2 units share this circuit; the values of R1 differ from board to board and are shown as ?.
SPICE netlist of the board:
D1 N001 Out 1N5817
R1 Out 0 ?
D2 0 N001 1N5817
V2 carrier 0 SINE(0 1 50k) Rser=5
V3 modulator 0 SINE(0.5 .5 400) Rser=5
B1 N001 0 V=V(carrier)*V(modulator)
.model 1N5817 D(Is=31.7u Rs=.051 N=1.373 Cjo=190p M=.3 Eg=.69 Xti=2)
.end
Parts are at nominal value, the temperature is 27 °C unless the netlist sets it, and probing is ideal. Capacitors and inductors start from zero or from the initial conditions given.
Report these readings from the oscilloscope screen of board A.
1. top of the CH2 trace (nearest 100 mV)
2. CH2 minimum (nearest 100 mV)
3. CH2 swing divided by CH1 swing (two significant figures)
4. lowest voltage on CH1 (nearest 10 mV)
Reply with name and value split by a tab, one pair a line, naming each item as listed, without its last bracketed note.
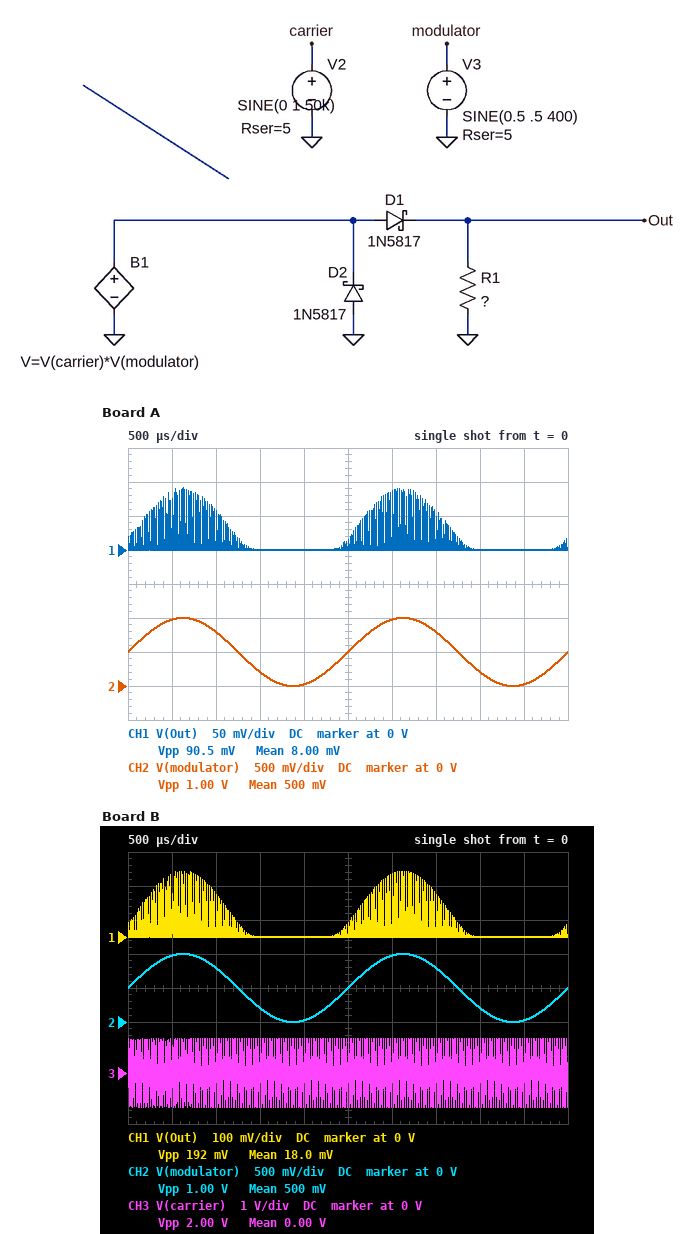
top of the CH2 trace	1.0 V
CH2 minimum	0 V
CH2 swing divided by CH1 swing	11
lowest voltage on CH1	0 V
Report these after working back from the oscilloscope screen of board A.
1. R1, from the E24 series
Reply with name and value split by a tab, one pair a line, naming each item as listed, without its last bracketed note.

R1, from the E24 series	0.01 Ω
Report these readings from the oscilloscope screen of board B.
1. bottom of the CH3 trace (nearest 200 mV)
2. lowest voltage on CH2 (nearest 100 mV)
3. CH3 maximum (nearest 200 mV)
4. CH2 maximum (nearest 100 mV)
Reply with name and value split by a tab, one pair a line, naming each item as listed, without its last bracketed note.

bottom of the CH3 trace	-1.0 V
lowest voltage on CH2	0 V
CH3 maximum	1.0 V
CH2 maximum	1.0 V
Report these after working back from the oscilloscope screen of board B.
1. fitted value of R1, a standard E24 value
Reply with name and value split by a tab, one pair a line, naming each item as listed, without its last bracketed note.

fitted value of R1, a standard E24 value	0.027 Ω
